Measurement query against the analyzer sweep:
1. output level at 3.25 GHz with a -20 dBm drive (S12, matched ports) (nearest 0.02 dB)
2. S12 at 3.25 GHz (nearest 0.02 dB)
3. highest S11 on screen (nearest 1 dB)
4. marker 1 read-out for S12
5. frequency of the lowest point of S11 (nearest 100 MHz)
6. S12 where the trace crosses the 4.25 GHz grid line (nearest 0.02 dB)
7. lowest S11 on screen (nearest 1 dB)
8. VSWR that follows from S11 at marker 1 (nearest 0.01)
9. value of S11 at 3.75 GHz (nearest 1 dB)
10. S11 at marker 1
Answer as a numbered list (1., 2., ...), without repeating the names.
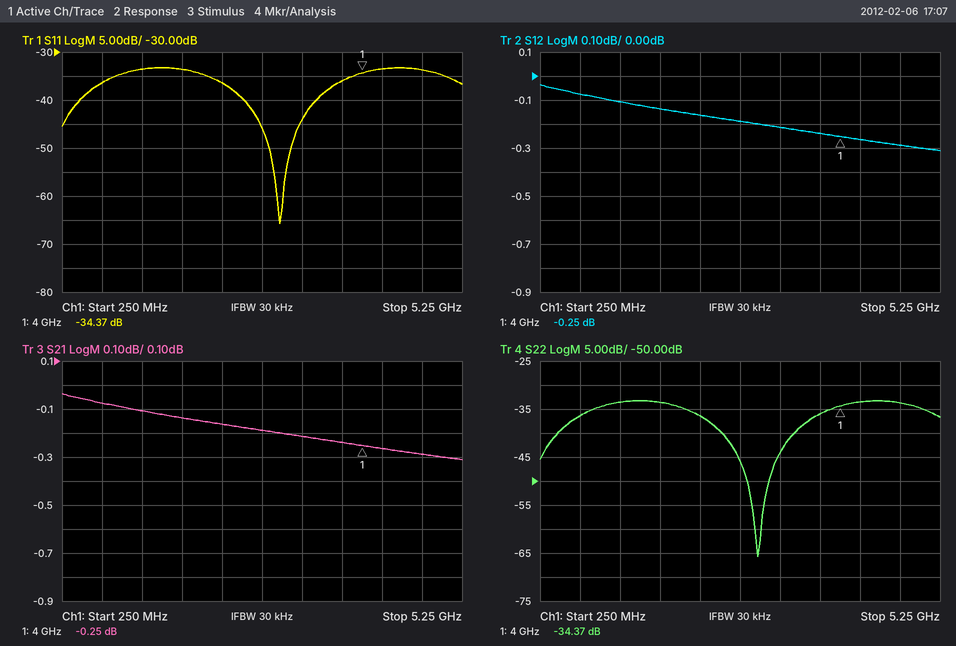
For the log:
1. -20.22 dBm
2. -0.22 dB
3. -33 dB
4. -0.25 dB
5. 3.0 GHz
6. -0.26 dB
7. -66 dB
8. 1.04
9. -36 dB
10. -34.37 dB
